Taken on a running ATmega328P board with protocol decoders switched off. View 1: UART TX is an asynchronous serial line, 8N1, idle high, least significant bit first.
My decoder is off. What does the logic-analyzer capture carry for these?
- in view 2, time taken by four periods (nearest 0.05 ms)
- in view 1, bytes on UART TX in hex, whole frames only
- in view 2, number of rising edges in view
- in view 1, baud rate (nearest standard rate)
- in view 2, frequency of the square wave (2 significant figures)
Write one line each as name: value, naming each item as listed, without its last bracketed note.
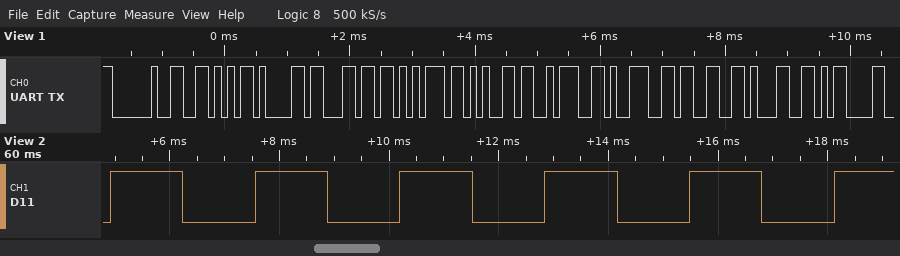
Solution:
in view 2, time taken by four periods: 10.55 ms
in view 1, bytes on UART TX in hex, whole frames only: 0x20 0x56 0x61 0x6C 0x75 0x65 0x3A 0x39 0x33 0x31 0x0D
in view 2, number of rising edges in view: 6
in view 1, baud rate: 9600 baud
in view 2, frequency of the square wave: 380 Hz
